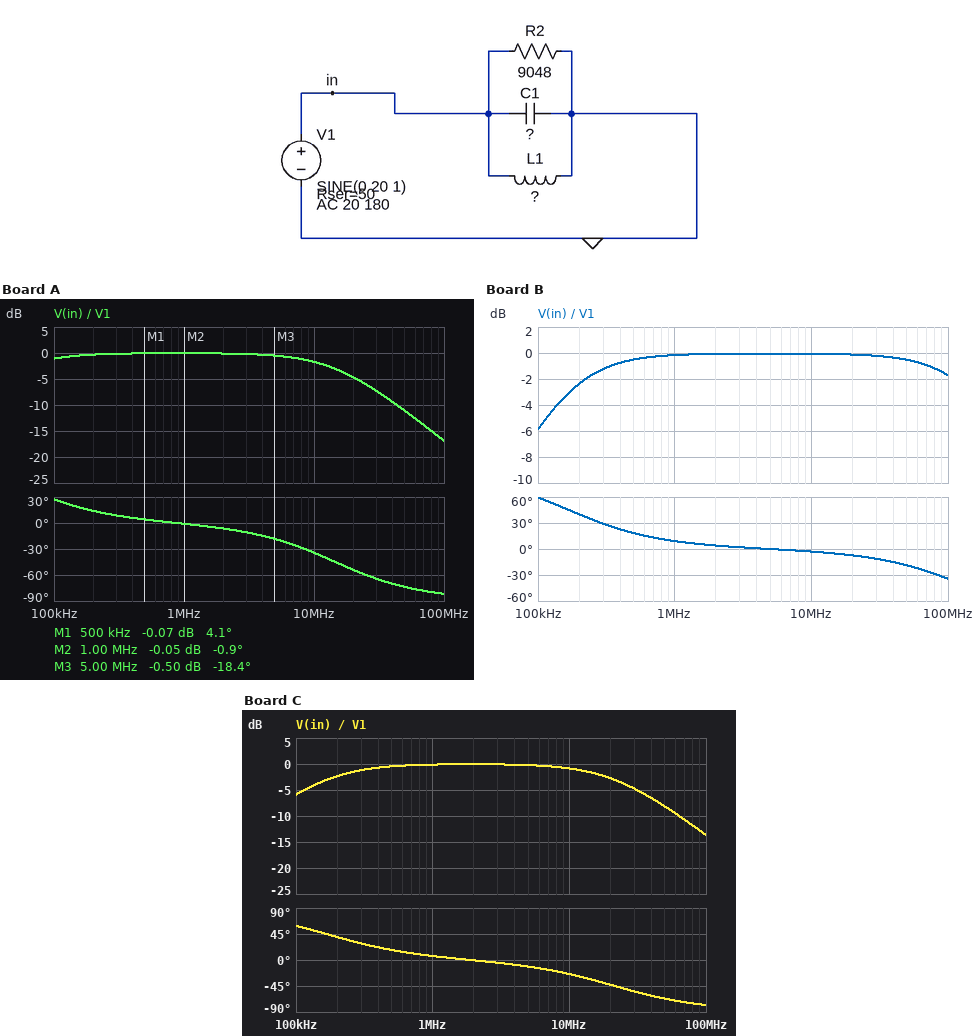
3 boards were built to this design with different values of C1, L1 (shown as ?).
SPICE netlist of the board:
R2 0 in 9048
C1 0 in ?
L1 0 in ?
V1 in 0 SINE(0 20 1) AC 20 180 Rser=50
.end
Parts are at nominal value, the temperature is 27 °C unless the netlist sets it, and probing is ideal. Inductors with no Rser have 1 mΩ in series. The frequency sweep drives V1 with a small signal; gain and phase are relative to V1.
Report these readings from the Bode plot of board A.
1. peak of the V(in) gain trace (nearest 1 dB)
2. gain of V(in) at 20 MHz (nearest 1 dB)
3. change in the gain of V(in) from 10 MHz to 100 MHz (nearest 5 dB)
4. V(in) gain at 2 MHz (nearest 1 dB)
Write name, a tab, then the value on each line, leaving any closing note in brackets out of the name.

peak of the V(in) gain trace	0 dB
gain of V(in) at 20 MHz	-5 dB
change in the gain of V(in) from 10 MHz to 100 MHz	-15 dB
V(in) gain at 2 MHz	0 dB
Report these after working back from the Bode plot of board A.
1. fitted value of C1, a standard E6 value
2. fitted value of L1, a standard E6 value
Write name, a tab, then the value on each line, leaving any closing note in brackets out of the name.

fitted value of C1, a standard E6 value	220 pF
fitted value of L1, a standard E6 value	150 µH
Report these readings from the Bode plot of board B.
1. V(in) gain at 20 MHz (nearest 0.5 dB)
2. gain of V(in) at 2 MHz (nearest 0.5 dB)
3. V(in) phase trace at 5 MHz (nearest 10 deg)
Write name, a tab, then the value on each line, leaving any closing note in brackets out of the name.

V(in) gain at 20 MHz	0 dB
gain of V(in) at 2 MHz	0 dB
V(in) phase trace at 5 MHz	0 deg
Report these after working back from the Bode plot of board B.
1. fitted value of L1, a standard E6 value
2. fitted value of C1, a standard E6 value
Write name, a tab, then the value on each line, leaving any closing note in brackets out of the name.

fitted value of L1, a standard E6 value	47 µH
fitted value of C1, a standard E6 value	22 pF
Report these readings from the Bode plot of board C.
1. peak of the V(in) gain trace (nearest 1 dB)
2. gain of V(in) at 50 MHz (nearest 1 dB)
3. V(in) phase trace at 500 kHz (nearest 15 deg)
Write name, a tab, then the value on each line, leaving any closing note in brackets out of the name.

peak of the V(in) gain trace	0 dB
gain of V(in) at 50 MHz	-8 dB
V(in) phase trace at 500 kHz	15 deg
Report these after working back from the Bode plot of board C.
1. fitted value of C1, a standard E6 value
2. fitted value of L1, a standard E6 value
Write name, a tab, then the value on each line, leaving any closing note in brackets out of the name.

fitted value of C1, a standard E6 value	150 pF
fitted value of L1, a standard E6 value	47 µH
